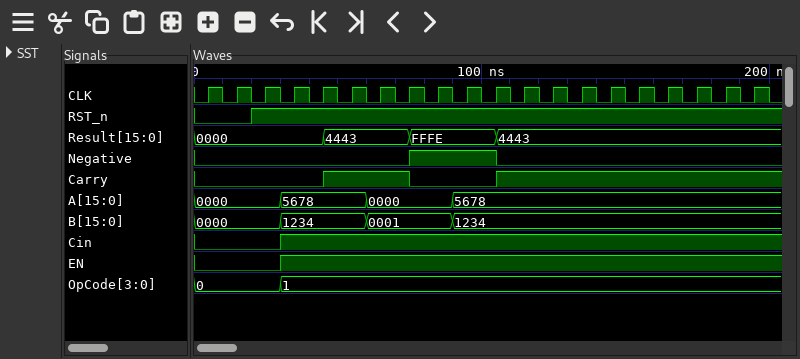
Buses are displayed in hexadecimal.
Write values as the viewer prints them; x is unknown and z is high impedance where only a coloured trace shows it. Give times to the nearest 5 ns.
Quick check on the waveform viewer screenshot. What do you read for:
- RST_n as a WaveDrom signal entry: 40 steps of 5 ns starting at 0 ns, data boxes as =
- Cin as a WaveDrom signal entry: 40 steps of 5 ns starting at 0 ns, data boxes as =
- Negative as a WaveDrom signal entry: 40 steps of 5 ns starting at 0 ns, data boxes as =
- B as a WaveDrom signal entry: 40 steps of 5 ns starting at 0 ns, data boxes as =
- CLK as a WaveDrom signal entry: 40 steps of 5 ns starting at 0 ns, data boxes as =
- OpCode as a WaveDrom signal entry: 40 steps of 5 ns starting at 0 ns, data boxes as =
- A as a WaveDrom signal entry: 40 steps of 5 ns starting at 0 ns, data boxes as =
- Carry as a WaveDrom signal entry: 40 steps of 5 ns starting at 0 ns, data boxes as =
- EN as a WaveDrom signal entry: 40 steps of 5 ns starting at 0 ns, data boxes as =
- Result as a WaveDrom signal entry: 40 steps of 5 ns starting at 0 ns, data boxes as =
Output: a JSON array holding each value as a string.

["{name: 'RST_n', wave: '0...1...................................'}", "{name: 'Cin', wave: '0.....1.................................'}", "{name: 'Negative', wave: '0..............1.....0..................'}", "{name: 'B', wave: '=.....=.....=.....=.....................', data: '0000 1234 0001 1234'}", "{name: 'CLK', wave: '0101010101010101010101010101010101010101'}", "{name: 'OpCode', wave: '=.....=.................................', data: '0 1'}", "{name: 'A', wave: '=.....=.....=.....=.....................', data: '0000 5678 0000 5678'}", "{name: 'Carry', wave: '0........1.....0.....1..................'}", "{name: 'EN', wave: '0.....1.................................'}", "{name: 'Result', wave: '=........=.....=.....=..................', data: '0000 4443 FFFE 4443'}"]
